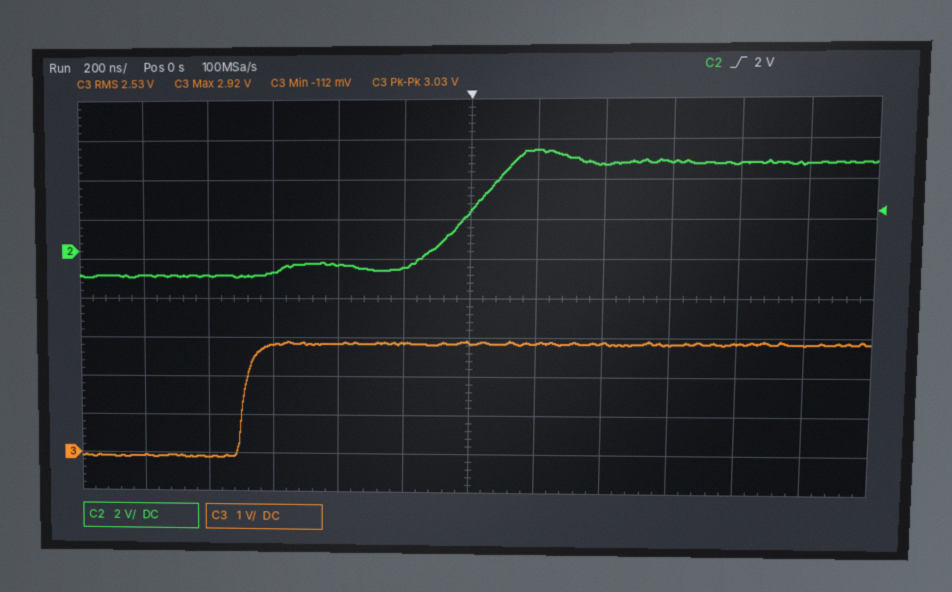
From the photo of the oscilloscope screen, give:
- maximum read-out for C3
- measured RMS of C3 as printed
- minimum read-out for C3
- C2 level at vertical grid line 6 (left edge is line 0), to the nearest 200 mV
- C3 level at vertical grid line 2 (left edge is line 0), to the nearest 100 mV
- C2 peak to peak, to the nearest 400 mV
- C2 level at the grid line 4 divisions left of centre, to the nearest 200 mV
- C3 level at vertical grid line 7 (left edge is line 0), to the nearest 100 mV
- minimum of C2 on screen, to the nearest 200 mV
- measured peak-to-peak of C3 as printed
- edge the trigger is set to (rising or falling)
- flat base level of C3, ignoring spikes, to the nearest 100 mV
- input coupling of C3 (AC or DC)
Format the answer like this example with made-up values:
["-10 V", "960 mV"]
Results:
["2.92 V", "2.53 V", "-112 mV", "2.0 V", "-100 mV", "6.4 V", "-1.2 V", "2.9 V", "-1.2 V", "3.03 V", "rising", "-100 mV", "DC"]
